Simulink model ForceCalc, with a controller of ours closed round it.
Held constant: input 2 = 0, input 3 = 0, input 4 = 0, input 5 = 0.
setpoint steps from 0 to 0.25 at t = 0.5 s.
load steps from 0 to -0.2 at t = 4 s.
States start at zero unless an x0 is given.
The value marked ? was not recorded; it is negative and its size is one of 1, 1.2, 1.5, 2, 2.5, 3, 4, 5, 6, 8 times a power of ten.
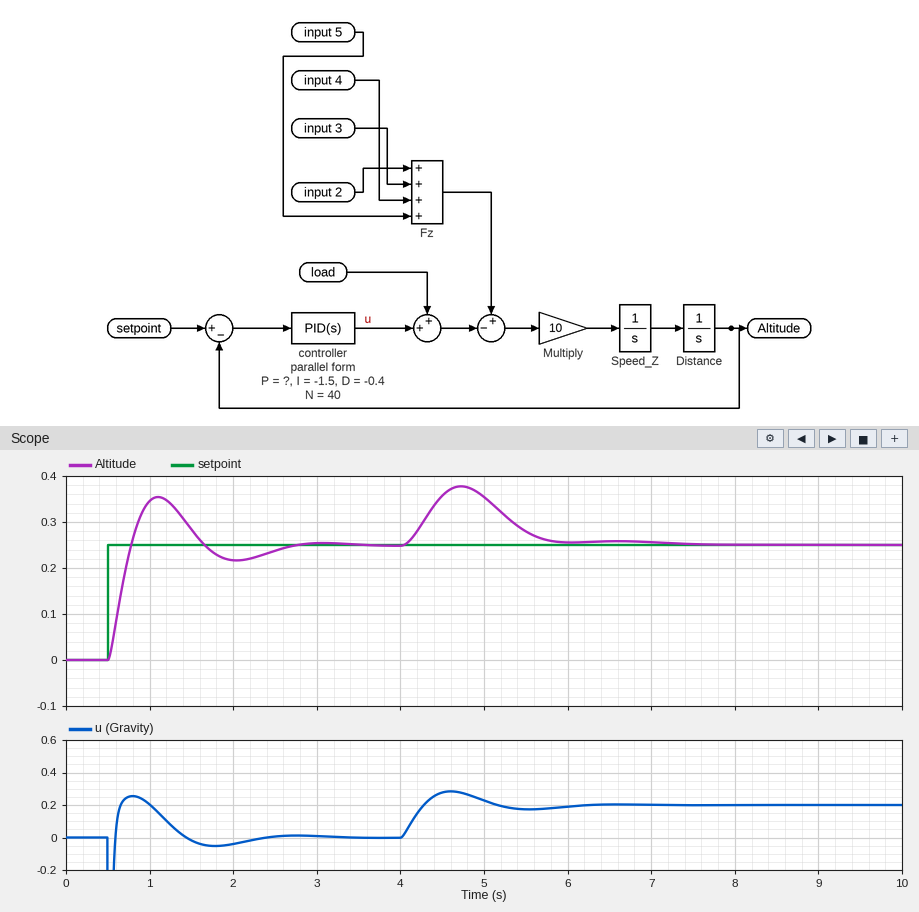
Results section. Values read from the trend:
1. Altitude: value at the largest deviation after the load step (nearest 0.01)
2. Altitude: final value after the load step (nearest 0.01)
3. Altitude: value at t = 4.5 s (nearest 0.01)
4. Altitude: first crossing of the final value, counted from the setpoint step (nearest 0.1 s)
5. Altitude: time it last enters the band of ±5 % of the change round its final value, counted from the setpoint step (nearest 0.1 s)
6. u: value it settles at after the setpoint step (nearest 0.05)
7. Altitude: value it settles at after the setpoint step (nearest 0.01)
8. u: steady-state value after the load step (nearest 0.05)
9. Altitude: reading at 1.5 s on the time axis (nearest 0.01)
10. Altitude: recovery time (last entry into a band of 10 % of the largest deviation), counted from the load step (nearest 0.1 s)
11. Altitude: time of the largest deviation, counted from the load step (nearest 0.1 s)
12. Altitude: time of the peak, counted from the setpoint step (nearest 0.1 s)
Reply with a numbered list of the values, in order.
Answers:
1. 0.38
2. 0.25
3. 0.36
4. 0.3 s
5. 2.0 s
6. 0.00
7. 0.25
8. 0.20
9. 0.28
10. 1.7 s
11. 0.7 s
12. 0.6 s
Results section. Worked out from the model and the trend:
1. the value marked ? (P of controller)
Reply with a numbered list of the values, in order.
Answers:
1. -1.5
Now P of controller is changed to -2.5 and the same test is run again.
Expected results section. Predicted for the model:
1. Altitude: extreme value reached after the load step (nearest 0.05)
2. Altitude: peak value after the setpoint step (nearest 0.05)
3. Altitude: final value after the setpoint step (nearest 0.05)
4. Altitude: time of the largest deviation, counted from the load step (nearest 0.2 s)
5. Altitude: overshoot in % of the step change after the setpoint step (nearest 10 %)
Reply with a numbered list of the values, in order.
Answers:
1. 0.35
2. 0.35
3. 0.25
4. 0.6 s
5. 50 %
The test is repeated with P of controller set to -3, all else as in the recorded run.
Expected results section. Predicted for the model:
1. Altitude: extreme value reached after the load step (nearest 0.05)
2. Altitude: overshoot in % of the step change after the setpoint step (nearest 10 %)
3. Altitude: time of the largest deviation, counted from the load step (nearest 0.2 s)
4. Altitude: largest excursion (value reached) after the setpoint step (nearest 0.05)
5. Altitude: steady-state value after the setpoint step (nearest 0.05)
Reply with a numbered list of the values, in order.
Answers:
1. 0.35
2. 50 %
3. 0.6 s
4. 0.35
5. 0.25
